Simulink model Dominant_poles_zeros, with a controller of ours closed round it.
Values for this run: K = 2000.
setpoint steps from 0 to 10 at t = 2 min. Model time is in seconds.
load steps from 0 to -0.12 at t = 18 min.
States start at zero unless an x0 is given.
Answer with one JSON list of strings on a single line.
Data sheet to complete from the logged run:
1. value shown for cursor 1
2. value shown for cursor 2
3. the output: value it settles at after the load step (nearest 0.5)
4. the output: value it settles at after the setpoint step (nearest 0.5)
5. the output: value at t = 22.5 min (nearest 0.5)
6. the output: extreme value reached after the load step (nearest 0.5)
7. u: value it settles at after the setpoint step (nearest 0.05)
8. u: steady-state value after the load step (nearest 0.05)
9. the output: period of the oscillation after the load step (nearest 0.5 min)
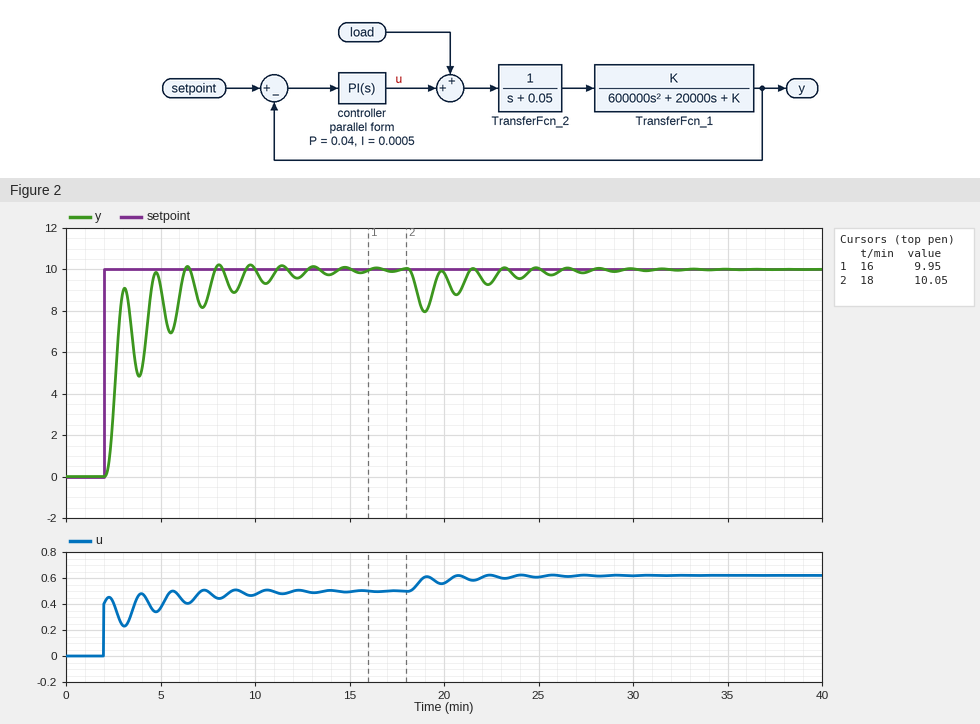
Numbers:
["9.95", "10.05", "10.0", "10.0", "9.5", "8.0", "0.50", "0.60", "1.5 min"]
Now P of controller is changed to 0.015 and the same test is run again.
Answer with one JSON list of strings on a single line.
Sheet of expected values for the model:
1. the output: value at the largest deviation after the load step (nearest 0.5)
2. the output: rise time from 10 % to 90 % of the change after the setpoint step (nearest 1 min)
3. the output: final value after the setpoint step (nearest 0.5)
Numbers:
["7.5", "4 min", "10.0"]
